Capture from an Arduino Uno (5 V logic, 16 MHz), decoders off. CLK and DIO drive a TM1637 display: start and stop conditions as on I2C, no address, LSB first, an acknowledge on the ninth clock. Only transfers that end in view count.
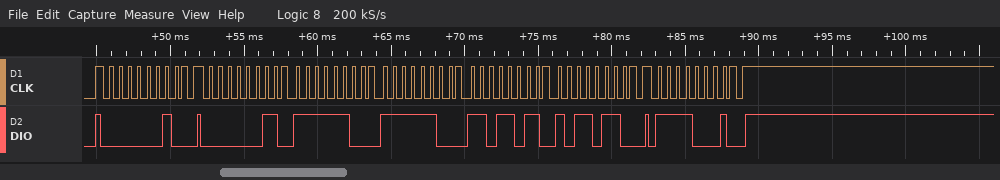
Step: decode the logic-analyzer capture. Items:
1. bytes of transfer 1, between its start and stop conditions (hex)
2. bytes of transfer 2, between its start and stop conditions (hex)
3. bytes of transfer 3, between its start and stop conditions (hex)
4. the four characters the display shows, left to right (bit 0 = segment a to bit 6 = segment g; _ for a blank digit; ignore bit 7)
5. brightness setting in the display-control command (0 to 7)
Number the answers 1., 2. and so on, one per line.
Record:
1. 40
2. C0 3F 3F DB 6D
3. 8F
4. 0025
5. 7
